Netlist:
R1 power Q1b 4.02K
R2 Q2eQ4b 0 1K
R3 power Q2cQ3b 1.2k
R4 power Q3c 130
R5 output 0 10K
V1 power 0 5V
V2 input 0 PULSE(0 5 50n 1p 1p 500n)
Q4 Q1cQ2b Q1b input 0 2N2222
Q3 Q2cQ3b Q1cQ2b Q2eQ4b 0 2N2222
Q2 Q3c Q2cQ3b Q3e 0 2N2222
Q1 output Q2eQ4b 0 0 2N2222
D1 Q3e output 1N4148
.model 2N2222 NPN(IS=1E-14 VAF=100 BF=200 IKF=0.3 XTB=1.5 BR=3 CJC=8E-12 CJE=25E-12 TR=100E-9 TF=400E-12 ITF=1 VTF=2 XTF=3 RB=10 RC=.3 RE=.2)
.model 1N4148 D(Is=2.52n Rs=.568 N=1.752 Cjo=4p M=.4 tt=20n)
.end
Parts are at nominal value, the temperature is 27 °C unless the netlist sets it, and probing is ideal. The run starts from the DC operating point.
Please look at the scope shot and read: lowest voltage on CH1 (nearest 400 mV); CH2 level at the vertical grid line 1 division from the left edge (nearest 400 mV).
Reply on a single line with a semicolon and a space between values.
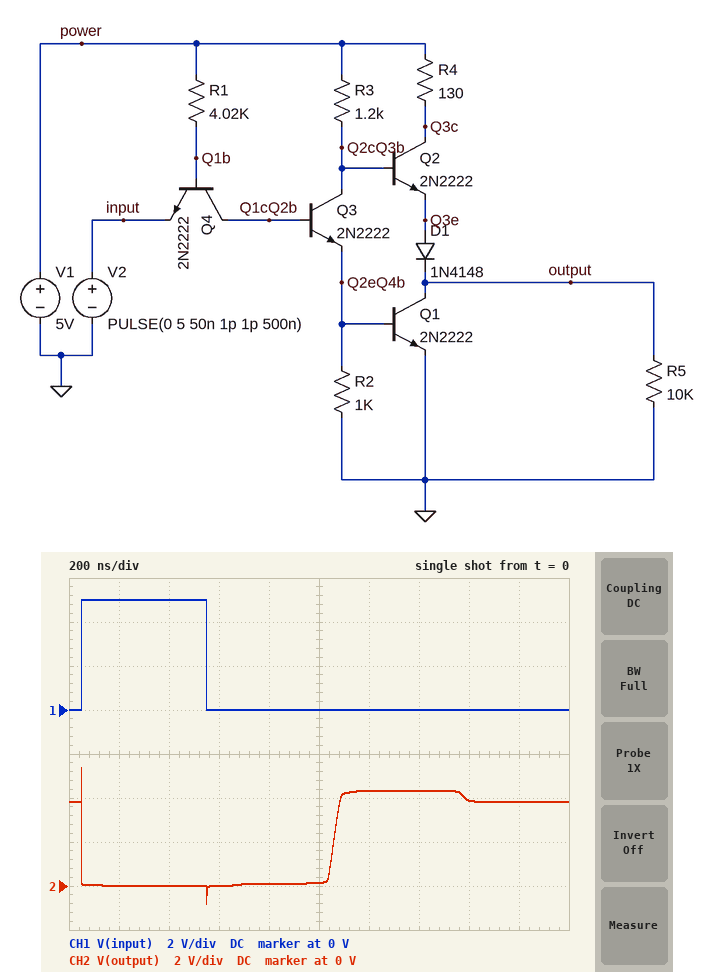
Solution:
0 V; 0 V
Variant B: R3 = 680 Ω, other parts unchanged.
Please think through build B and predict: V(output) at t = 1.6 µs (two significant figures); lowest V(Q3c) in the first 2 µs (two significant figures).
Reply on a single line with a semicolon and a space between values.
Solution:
4.3 V; 910 mV
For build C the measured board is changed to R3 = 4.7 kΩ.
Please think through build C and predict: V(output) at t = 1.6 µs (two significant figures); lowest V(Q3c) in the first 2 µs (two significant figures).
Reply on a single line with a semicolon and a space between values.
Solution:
3.8 V; 1.6 V
